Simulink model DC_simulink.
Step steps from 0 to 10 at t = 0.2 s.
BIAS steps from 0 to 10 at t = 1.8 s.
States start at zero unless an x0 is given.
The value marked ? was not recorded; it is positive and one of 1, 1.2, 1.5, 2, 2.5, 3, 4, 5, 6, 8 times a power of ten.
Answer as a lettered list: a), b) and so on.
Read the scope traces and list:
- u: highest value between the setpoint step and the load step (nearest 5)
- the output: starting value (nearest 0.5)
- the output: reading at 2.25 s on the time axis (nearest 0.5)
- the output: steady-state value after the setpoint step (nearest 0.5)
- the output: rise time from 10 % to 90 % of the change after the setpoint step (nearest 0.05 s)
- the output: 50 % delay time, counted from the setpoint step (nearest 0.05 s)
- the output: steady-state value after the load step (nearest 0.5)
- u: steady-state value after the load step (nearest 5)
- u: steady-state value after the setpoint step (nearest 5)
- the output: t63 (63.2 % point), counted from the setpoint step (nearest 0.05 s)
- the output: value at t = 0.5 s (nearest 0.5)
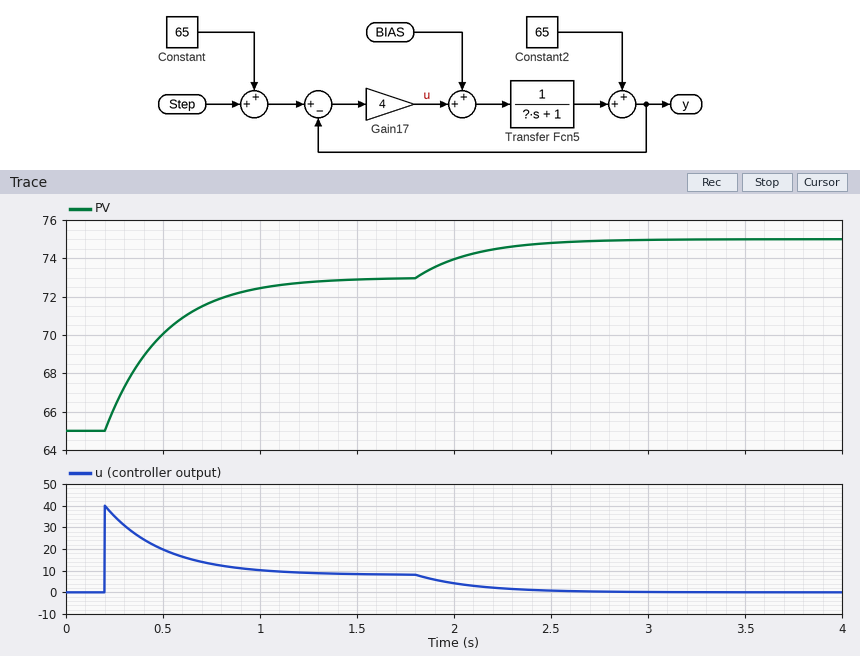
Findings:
a) 40
b) 65.0
c) 74.5
d) 73.0
e) 0.65 s
f) 0.20 s
g) 75.0
h) 0
i) 10
j) 0.30 s
k) 70.0
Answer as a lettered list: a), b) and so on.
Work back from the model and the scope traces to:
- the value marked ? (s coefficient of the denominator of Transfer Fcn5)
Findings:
a) 1.5
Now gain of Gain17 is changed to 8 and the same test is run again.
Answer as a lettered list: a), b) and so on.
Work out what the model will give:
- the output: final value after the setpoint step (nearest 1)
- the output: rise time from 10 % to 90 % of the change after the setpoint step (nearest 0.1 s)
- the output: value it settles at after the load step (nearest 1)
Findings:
a) 74
b) 0.4 s
c) 75
